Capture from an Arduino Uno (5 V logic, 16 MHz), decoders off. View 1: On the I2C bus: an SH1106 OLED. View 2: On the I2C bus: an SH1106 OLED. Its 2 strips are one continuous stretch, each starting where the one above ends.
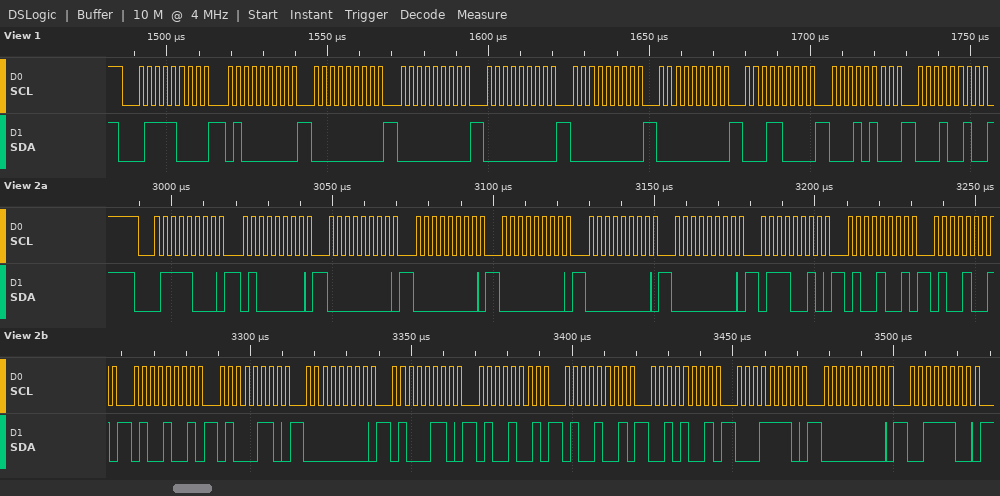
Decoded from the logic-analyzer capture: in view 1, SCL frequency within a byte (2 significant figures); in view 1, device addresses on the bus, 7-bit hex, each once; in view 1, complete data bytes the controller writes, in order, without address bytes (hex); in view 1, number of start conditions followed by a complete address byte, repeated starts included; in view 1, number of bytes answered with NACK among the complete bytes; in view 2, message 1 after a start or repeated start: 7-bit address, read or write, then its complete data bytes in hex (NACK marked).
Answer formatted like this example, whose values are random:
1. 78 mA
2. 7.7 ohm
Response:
1. 400 kHz
2. 0x3C
3. 40 00 00 00 00 00 18 14 12
4. 1
5. 0
6. 0x3C write: 40 00 00 00 00 00 72 49 49 49 46 00 46 49 49 29 1E 00 3C
